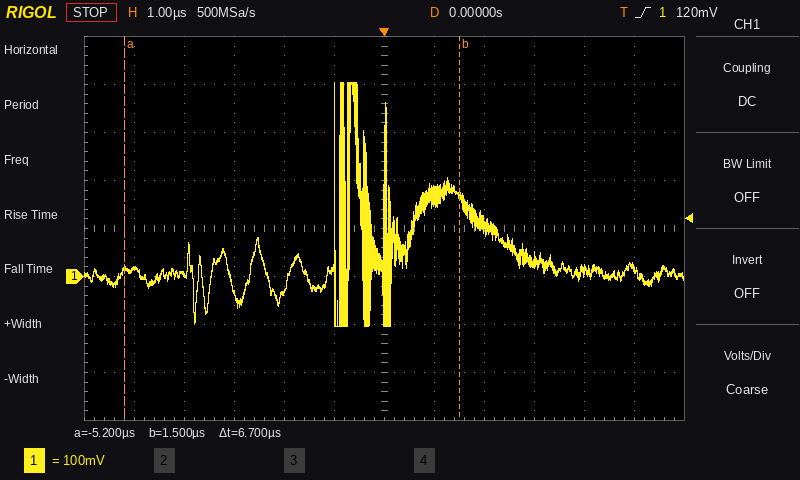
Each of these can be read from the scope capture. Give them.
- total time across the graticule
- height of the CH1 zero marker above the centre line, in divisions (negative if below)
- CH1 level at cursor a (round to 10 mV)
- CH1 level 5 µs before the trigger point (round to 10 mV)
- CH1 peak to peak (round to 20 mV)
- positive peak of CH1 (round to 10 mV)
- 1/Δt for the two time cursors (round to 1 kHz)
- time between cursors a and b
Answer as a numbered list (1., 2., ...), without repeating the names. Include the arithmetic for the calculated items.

1. 12 µs
2. -1.0 div
3. 10 mV
4. 10 mV
5. 500 mV
6. 400 mV
7. 1 / 6.7 µs ≈ 149 kHz
8. 6.7 µs
